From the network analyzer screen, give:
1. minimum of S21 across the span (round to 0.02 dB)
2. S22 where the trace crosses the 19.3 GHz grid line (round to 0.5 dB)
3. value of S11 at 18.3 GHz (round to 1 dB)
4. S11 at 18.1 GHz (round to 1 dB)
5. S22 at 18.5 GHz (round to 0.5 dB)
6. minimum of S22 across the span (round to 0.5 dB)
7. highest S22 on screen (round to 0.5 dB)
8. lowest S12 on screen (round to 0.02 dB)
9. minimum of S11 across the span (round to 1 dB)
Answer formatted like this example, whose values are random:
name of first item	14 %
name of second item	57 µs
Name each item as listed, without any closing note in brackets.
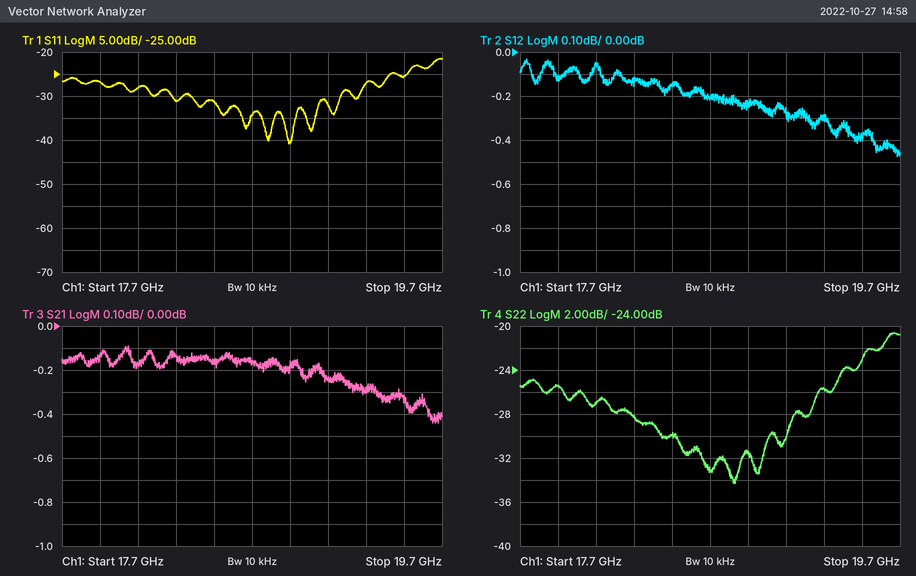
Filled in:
minimum of S21 across the span	-0.44 dB
S22 where the trace crosses the 19.3 GHz grid line	-25.5 dB
value of S11 at 18.3 GHz	-31 dB
S11 at 18.1 GHz	-28 dB
S22 at 18.5 GHz	-30.0 dB
minimum of S22 across the span	-34.5 dB
highest S22 on screen	-20.5 dB
lowest S12 on screen	-0.48 dB
minimum of S11 across the span	-41 dB
